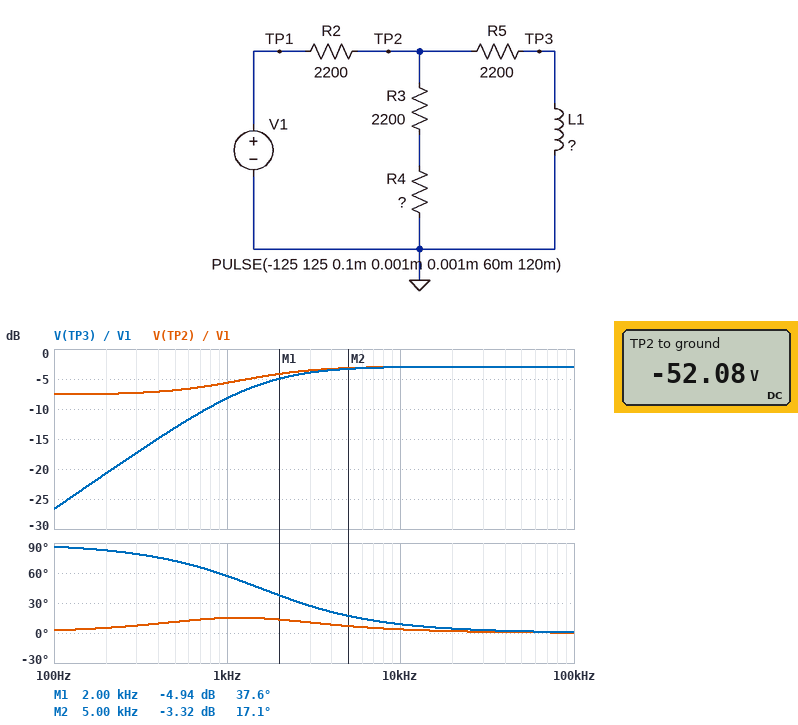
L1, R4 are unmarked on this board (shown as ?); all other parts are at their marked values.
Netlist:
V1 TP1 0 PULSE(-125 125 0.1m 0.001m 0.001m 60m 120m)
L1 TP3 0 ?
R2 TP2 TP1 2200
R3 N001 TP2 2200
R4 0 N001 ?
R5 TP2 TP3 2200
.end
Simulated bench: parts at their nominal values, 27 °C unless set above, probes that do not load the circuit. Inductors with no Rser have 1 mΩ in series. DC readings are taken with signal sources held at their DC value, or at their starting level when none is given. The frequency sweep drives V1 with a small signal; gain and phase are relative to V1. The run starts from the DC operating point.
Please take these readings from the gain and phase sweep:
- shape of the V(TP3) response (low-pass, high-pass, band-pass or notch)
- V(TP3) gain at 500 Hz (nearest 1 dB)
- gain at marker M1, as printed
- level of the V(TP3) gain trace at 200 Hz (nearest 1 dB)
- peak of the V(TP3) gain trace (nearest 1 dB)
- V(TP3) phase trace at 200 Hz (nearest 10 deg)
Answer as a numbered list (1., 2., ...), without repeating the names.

1. high-pass
2. -13 dB
3. -4.94 dB
4. -21 dB
5. -3 dB
6. 80 deg
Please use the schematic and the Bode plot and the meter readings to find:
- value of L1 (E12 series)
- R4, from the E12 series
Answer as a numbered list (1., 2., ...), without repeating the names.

1. 390 mH
2. 3.3 kΩ
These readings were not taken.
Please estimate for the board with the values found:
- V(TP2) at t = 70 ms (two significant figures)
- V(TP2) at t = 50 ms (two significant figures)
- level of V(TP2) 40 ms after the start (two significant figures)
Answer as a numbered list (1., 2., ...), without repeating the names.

1. -52 V
2. 52 V
3. 52 V
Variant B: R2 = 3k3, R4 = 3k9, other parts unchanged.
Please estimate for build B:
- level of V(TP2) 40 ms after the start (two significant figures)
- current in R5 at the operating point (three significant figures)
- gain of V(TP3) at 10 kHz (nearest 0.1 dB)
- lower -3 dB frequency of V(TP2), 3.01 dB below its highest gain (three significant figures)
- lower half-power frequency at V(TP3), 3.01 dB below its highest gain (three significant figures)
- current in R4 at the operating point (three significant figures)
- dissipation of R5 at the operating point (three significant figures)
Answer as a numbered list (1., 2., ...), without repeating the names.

1. 41 V
2. 18.7 mA
3. -3.9 dB
4. 1.24 kHz
5. 1.77 kHz
6. 6.74 mA
7. 768 mW
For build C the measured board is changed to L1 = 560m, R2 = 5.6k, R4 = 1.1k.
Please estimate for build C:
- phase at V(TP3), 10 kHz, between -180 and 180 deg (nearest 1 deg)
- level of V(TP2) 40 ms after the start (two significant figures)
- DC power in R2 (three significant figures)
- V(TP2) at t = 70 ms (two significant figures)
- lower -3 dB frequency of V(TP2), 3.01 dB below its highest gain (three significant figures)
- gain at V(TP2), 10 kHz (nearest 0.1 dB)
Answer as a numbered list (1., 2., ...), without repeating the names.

1. 7 deg
2. 24 V
3. 1.83 W
4. -24 V
5. 834 Hz
6. -8.7 dB
